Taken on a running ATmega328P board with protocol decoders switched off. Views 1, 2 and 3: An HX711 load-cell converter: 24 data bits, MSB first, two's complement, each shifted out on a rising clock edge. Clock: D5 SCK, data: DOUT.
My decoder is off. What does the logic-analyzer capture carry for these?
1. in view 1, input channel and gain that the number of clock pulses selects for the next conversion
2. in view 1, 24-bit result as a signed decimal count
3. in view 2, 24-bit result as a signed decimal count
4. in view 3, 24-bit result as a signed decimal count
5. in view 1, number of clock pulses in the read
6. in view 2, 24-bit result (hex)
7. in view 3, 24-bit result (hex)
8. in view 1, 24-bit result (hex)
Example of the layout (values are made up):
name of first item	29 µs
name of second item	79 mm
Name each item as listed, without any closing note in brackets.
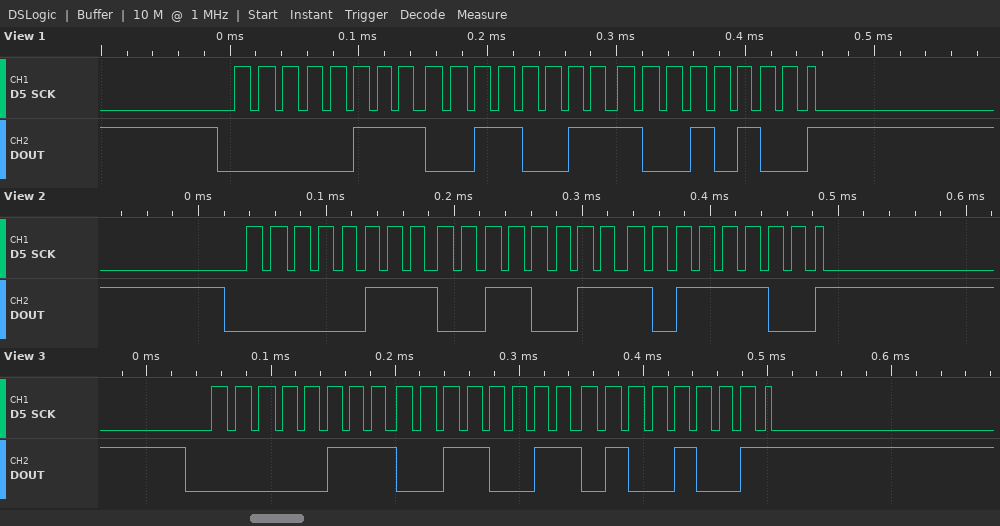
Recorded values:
in view 1, input channel and gain that the number of clock pulses selects for the next conversion	channel A, gain 128
in view 1, 24-bit result as a signed decimal count	471956
in view 2, 24-bit result as a signed decimal count	471996
in view 3, 24-bit result as a signed decimal count	471881
in view 1, number of clock pulses in the read	25
in view 2, 24-bit result	0x0733BC
in view 3, 24-bit result	0x073349
in view 1, 24-bit result	0x073394
